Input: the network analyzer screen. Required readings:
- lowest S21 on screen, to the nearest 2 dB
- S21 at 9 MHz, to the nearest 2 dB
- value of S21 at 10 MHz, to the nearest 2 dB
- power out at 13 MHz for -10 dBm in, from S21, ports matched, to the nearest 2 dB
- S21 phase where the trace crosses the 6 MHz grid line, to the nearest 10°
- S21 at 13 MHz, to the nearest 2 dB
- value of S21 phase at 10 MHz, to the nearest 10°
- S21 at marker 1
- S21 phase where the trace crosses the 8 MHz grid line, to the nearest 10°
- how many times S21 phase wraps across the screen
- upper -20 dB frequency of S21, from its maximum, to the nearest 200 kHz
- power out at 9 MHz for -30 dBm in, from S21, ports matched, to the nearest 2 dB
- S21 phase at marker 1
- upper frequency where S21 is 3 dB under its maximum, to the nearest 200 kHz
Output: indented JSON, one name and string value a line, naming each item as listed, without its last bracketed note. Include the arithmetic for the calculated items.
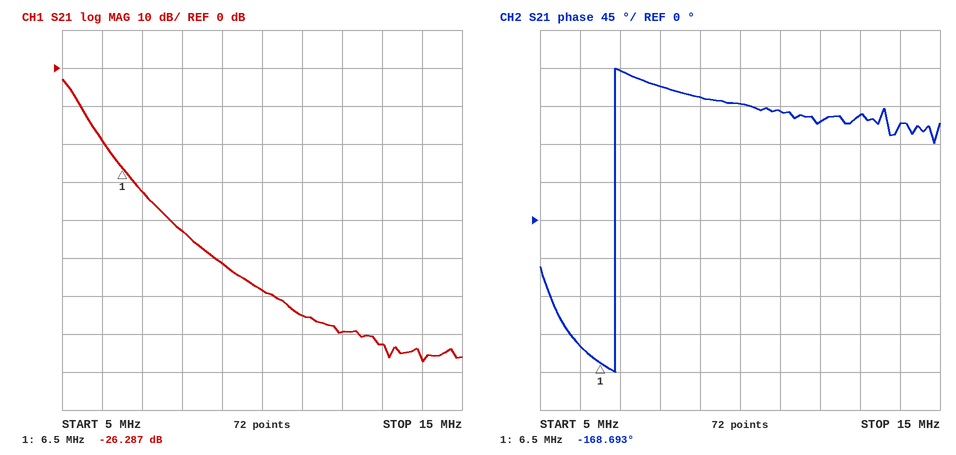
{
  "lowest S21 on screen, to the nearest 2 dB": "-78 dB",
  "S21 at 9 MHz, to the nearest 2 dB": "-52 dB",
  "value of S21 at 10 MHz, to the nearest 2 dB": "-58 dB",
  "power out at 13 MHz for -10 dBm in, from S21, ports matched, to the nearest 2 dB": "-10 dBm + (-72 dB) = -82 dBm",
  "S21 phase where the trace crosses the 6 MHz grid line, to the nearest 10°": "-150°",
  "S21 at 13 MHz, to the nearest 2 dB": "-72 dB",
  "value of S21 phase at 10 MHz, to the nearest 10°": "140°",
  "S21 at marker 1": "-26.287 dB",
  "S21 phase where the trace crosses the 8 MHz grid line, to the nearest 10°": "160°",
  "how many times S21 phase wraps across the screen": "1",
  "upper -20 dB frequency of S21, from its maximum, to the nearest 200 kHz": "6.2 MHz",
  "power out at 9 MHz for -30 dBm in, from S21, ports matched, to the nearest 2 dB": "-30 dBm + (-52 dB) = -82 dBm",
  "S21 phase at marker 1": "-168.693°",
  "upper frequency where S21 is 3 dB under its maximum, to the nearest 200 kHz": "5.2 MHz"
}
